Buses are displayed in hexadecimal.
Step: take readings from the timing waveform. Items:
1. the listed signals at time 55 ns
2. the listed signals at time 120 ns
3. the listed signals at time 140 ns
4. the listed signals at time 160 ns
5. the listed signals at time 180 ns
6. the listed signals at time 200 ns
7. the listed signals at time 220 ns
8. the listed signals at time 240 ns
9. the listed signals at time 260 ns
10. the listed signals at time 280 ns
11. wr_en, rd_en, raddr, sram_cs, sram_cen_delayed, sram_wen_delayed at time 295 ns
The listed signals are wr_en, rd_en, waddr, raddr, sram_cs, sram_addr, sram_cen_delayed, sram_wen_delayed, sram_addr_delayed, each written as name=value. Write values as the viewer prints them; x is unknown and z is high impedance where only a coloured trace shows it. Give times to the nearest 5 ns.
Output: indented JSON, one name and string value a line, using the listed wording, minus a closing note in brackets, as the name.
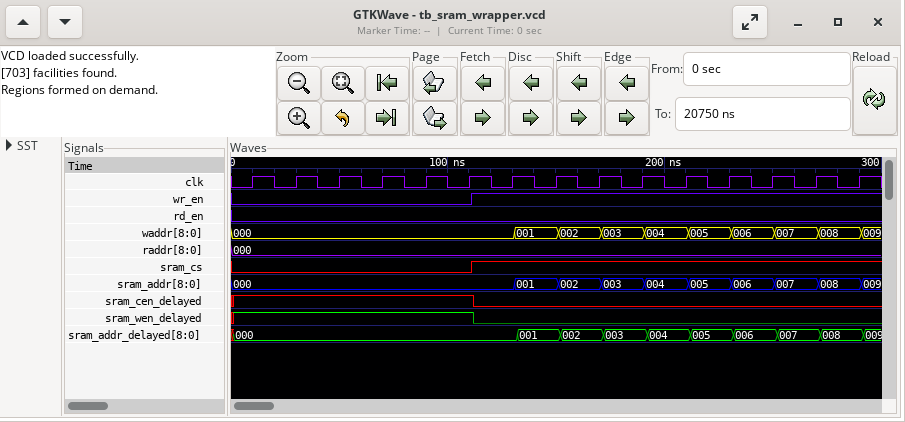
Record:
{
  "the listed signals at time 55 ns": "wr_en=0, rd_en=0, waddr=000, raddr=000, sram_cs=0, sram_addr=000, sram_cen_delayed=1, sram_wen_delayed=1, sram_addr_delayed=000",
  "the listed signals at time 120 ns": "wr_en=1, rd_en=0, waddr=000, raddr=000, sram_cs=1, sram_addr=000, sram_cen_delayed=0, sram_wen_delayed=0, sram_addr_delayed=000",
  "the listed signals at time 140 ns": "wr_en=1, rd_en=0, waddr=001, raddr=000, sram_cs=1, sram_addr=001, sram_cen_delayed=0, sram_wen_delayed=0, sram_addr_delayed=001",
  "the listed signals at time 160 ns": "wr_en=1, rd_en=0, waddr=002, raddr=000, sram_cs=1, sram_addr=002, sram_cen_delayed=0, sram_wen_delayed=0, sram_addr_delayed=002",
  "the listed signals at time 180 ns": "wr_en=1, rd_en=0, waddr=003, raddr=000, sram_cs=1, sram_addr=003, sram_cen_delayed=0, sram_wen_delayed=0, sram_addr_delayed=003",
  "the listed signals at time 200 ns": "wr_en=1, rd_en=0, waddr=004, raddr=000, sram_cs=1, sram_addr=004, sram_cen_delayed=0, sram_wen_delayed=0, sram_addr_delayed=004",
  "the listed signals at time 220 ns": "wr_en=1, rd_en=0, waddr=005, raddr=000, sram_cs=1, sram_addr=005, sram_cen_delayed=0, sram_wen_delayed=0, sram_addr_delayed=005",
  "the listed signals at time 240 ns": "wr_en=1, rd_en=0, waddr=006, raddr=000, sram_cs=1, sram_addr=006, sram_cen_delayed=0, sram_wen_delayed=0, sram_addr_delayed=006",
  "the listed signals at time 260 ns": "wr_en=1, rd_en=0, waddr=007, raddr=000, sram_cs=1, sram_addr=007, sram_cen_delayed=0, sram_wen_delayed=0, sram_addr_delayed=007",
  "the listed signals at time 280 ns": "wr_en=1, rd_en=0, waddr=008, raddr=000, sram_cs=1, sram_addr=008, sram_cen_delayed=0, sram_wen_delayed=0, sram_addr_delayed=008",
  "wr_en, rd_en, raddr, sram_cs, sram_cen_delayed, sram_wen_delayed at time 295 ns": "wr_en=1, rd_en=0, raddr=000, sram_cs=1, sram_cen_delayed=0, sram_wen_delayed=0"
}
